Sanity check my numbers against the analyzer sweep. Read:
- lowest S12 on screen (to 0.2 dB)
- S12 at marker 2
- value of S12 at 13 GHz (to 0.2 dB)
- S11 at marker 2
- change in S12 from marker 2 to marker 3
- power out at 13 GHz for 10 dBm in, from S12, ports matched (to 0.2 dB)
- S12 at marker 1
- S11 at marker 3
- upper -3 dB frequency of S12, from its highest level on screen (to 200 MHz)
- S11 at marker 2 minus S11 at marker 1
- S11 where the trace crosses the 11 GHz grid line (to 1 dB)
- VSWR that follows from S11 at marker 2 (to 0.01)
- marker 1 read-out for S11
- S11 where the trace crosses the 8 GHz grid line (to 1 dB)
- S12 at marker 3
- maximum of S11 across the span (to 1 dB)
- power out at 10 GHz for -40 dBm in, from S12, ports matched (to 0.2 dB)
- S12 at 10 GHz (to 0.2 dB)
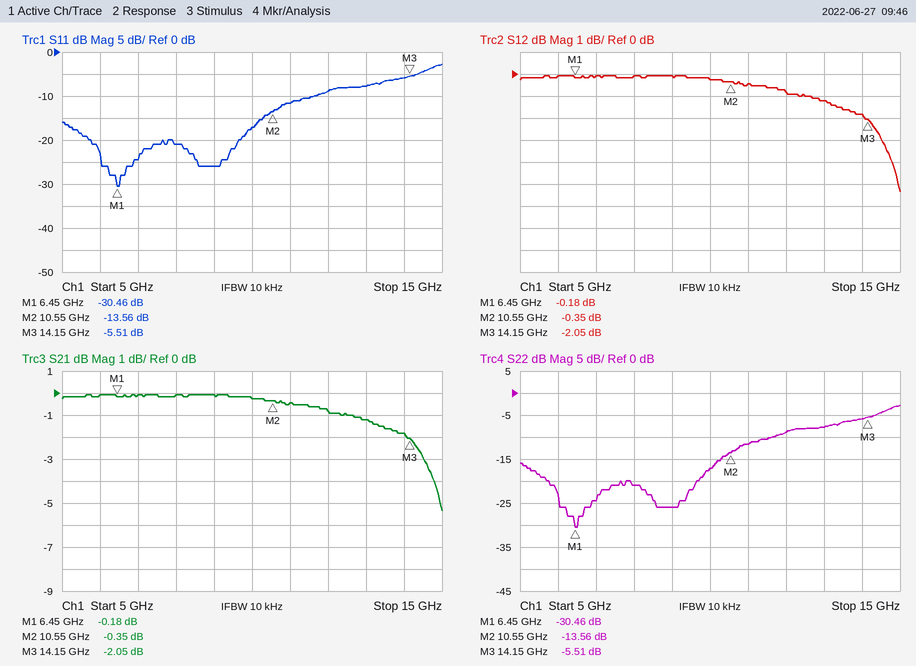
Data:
-5.4 dB
-0.35 dB
-1.2 dB
-13.56 dB
-1.70 dB
8.8 dBm
-0.18 dB
-5.51 dB
14.6 GHz
16.90 dB
-12 dB
1.53
-30.46 dB
-21 dB
-2.05 dB
-3 dB
-40.2 dBm
-0.2 dB
